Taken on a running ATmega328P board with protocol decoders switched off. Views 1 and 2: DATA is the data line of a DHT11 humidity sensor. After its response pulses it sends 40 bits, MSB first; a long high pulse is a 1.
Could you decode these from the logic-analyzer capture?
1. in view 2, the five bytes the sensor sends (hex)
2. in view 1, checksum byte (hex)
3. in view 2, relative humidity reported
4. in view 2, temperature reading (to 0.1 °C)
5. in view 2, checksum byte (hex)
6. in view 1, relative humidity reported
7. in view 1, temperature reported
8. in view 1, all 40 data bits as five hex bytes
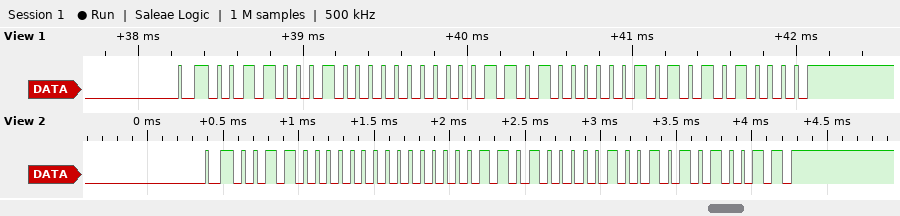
30 00 1A 09 53
0x50
48 %
26.9 °C
0x53
49 %
26.5 °C
31 00 1A 05 50
